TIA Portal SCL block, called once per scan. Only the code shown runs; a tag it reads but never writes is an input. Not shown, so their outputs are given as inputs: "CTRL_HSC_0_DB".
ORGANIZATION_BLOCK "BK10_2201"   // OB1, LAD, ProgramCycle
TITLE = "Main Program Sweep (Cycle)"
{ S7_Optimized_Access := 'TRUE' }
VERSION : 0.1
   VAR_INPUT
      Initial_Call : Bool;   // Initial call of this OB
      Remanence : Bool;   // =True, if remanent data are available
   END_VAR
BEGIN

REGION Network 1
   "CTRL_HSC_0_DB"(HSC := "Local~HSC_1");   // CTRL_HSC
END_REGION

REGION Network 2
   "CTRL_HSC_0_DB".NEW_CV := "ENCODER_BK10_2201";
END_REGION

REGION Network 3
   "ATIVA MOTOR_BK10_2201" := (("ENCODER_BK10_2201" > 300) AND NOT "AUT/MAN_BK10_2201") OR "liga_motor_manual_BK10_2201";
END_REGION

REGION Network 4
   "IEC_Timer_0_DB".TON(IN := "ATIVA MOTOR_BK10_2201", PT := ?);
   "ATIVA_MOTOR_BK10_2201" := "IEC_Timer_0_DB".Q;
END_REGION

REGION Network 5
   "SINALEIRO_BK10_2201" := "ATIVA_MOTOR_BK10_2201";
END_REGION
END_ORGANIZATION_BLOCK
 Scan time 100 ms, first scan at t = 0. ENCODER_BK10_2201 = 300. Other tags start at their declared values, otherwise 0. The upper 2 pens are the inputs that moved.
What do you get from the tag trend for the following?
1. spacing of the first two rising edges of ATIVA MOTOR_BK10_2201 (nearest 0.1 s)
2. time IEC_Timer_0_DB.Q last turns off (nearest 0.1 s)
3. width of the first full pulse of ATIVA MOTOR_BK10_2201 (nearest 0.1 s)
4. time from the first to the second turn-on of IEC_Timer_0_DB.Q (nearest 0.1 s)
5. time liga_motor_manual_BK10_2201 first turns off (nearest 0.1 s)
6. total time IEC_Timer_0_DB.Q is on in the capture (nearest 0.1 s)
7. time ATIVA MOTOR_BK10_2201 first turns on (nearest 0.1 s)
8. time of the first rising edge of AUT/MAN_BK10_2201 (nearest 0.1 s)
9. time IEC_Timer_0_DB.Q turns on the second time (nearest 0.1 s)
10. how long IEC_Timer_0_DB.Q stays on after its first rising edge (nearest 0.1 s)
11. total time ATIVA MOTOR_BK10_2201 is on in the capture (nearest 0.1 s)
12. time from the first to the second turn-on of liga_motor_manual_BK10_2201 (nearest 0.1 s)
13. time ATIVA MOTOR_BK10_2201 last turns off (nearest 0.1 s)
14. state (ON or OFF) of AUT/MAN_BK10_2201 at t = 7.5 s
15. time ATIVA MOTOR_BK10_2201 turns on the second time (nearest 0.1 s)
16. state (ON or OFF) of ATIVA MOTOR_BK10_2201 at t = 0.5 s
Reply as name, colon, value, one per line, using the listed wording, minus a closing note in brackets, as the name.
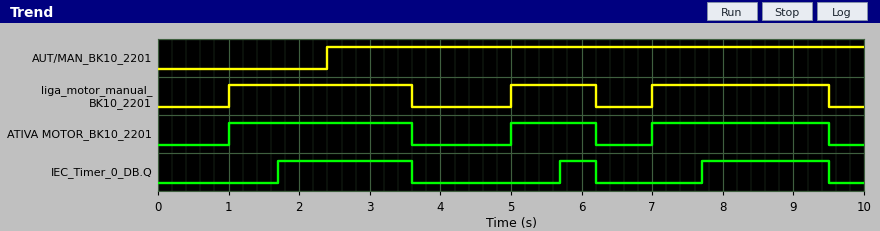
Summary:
spacing of the first two rising edges of ATIVA MOTOR_BK10_2201: 4.0 s
time IEC_Timer_0_DB.Q last turns off: 9.5 s
width of the first full pulse of ATIVA MOTOR_BK10_2201: 2.6 s
time from the first to the second turn-on of IEC_Timer_0_DB.Q: 4.0 s
time liga_motor_manual_BK10_2201 first turns off: 3.6 s
total time IEC_Timer_0_DB.Q is on in the capture: 4.2 s
time ATIVA MOTOR_BK10_2201 first turns on: 1.0 s
time of the first rising edge of AUT/MAN_BK10_2201: 2.4 s
time IEC_Timer_0_DB.Q turns on the second time: 5.7 s
how long IEC_Timer_0_DB.Q stays on after its first rising edge: 1.9 s
total time ATIVA MOTOR_BK10_2201 is on in the capture: 6.3 s
time from the first to the second turn-on of liga_motor_manual_BK10_2201: 4.0 s
time ATIVA MOTOR_BK10_2201 last turns off: 9.5 s
state (ON or OFF) of AUT/MAN_BK10_2201 at t = 7.5 s: ON
time ATIVA MOTOR_BK10_2201 turns on the second time: 5.0 s
state (ON or OFF) of ATIVA MOTOR_BK10_2201 at t = 0.5 s: OFF
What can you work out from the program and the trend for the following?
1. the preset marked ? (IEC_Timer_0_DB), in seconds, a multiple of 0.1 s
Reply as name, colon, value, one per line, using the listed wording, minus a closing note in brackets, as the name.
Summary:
the preset marked ? (IEC_Timer_0_DB), in seconds, a multiple of 0.1 s: 0.7 s
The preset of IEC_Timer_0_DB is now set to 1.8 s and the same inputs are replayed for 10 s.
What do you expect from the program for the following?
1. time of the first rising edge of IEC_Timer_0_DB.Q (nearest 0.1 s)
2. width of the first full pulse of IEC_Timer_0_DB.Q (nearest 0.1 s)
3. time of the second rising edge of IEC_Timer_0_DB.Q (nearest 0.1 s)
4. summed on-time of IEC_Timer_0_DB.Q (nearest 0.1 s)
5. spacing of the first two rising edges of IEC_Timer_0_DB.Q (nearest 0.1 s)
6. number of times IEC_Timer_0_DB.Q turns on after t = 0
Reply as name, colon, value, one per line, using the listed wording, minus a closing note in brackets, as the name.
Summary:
time of the first rising edge of IEC_Timer_0_DB.Q: 2.8 s
width of the first full pulse of IEC_Timer_0_DB.Q: 0.8 s
time of the second rising edge of IEC_Timer_0_DB.Q: 8.8 s
summed on-time of IEC_Timer_0_DB.Q: 1.5 s
spacing of the first two rising edges of IEC_Timer_0_DB.Q: 6.0 s
number of times IEC_Timer_0_DB.Q turns on after t = 0: 2
